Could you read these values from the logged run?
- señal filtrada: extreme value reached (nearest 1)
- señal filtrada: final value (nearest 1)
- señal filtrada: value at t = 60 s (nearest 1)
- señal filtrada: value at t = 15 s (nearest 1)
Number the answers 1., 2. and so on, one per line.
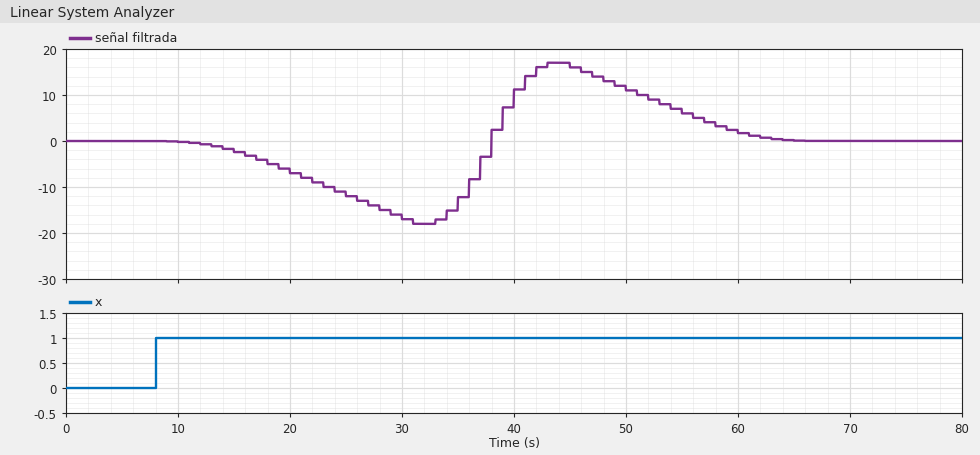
1. -18
2. 0
3. 2
4. -2
